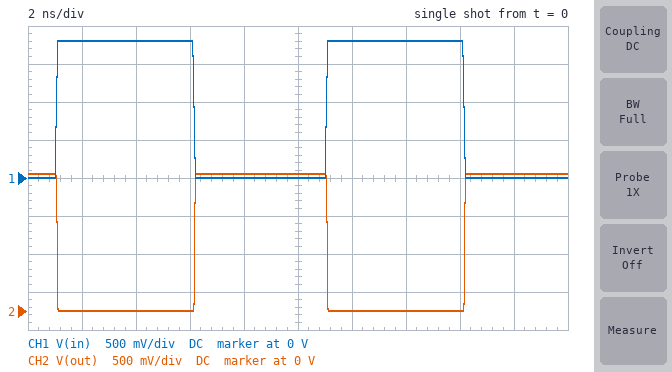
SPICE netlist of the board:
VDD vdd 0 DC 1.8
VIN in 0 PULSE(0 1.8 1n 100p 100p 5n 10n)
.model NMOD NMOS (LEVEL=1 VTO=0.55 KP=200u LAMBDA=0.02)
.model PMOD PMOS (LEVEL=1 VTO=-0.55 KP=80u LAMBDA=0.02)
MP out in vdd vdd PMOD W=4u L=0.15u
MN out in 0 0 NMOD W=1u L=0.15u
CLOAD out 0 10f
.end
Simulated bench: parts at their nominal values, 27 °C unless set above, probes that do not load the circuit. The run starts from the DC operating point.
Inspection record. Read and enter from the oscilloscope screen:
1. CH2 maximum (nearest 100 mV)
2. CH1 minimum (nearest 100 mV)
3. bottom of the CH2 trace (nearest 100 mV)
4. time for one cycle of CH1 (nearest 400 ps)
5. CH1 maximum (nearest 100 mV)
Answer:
1.8 V
0 V
0 V
10.0 ns
1.8 V
